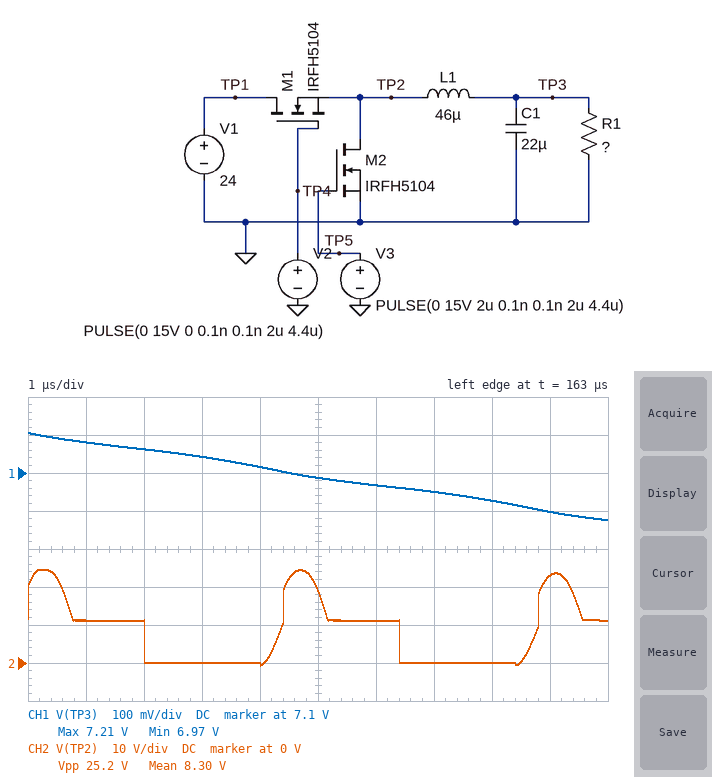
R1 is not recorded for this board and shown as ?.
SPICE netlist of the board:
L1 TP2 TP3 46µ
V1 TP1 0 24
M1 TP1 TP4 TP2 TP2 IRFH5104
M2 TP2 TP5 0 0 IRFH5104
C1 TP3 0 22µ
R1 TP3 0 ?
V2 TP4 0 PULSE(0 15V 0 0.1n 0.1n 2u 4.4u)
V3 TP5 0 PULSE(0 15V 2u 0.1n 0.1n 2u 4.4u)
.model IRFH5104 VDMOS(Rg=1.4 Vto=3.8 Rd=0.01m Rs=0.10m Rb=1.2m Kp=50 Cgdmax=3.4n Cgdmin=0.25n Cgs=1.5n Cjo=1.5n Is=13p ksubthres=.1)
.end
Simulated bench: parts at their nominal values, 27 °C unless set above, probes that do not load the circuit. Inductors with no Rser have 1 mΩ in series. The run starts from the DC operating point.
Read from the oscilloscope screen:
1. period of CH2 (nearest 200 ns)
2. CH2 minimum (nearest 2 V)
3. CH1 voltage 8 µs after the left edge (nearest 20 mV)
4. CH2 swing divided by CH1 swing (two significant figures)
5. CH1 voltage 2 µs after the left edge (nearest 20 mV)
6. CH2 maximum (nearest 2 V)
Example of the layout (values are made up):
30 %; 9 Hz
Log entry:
4.4 µs; 0 V; 7.02 V; 110; 7.16 V; 24 V
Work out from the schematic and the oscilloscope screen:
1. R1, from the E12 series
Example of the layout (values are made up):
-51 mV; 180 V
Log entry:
12 Ω
